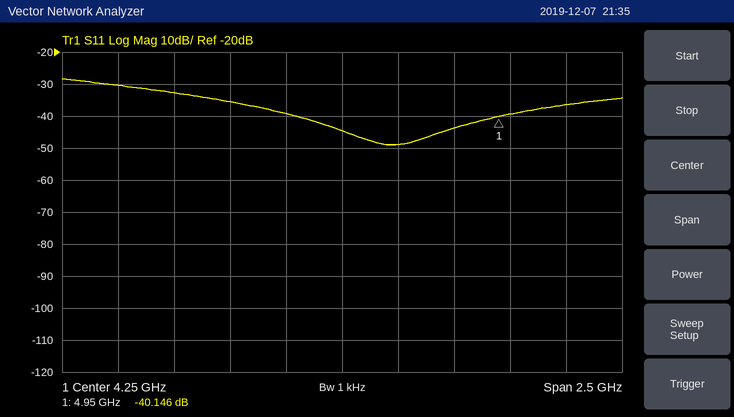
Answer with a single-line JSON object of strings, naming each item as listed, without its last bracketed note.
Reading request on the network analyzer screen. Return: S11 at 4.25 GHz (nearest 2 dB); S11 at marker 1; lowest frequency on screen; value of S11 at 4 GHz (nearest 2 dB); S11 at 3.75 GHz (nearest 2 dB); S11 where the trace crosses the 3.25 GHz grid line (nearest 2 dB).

{"S11 at 4.25 GHz": "-44 dB", "S11 at marker 1": "-40.146 dB", "lowest frequency on screen": "3 GHz", "value of S11 at 4 GHz": "-40 dB", "S11 at 3.75 GHz": "-36 dB", "S11 where the trace crosses the 3.25 GHz grid line": "-30 dB"}
